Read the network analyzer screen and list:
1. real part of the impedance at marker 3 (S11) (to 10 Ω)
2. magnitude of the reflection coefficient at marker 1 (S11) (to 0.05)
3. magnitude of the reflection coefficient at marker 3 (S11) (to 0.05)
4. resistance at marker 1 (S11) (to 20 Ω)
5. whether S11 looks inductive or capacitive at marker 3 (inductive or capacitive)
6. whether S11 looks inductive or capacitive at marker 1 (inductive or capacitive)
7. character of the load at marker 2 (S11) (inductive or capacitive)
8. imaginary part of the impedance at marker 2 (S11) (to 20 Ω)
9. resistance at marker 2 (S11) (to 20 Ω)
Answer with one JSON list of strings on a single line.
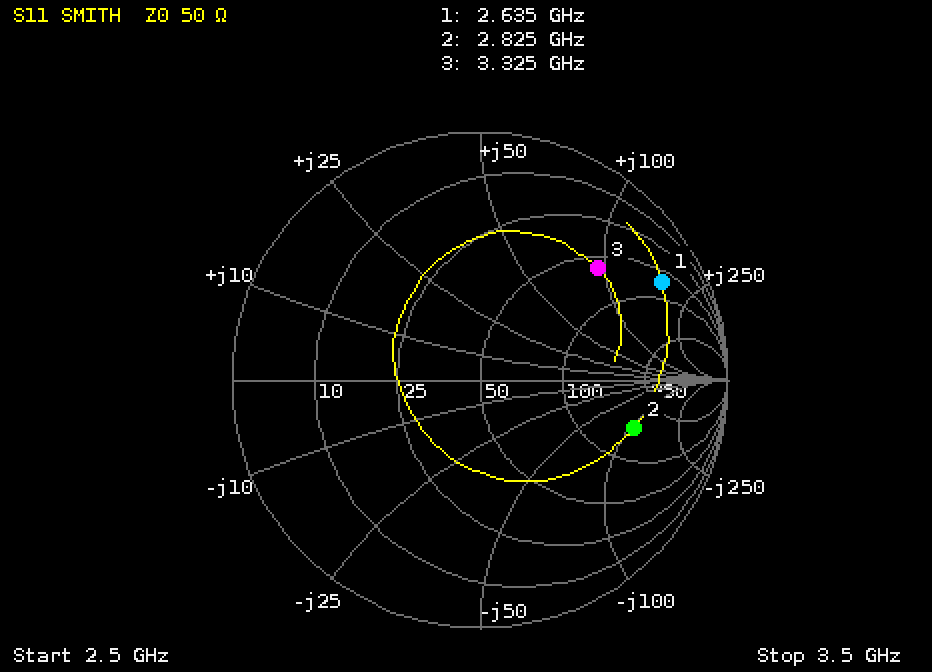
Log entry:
["60 Ω", "0.85", "0.65", "60 Ω", "inductive", "inductive", "capacitive", "-100 Ω", "160 Ω"]
